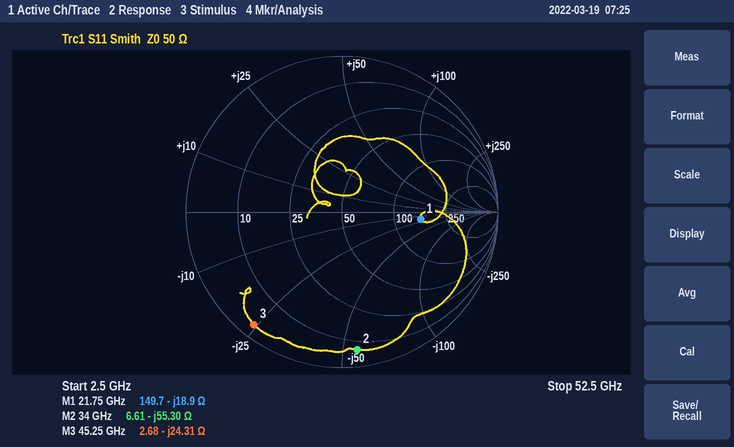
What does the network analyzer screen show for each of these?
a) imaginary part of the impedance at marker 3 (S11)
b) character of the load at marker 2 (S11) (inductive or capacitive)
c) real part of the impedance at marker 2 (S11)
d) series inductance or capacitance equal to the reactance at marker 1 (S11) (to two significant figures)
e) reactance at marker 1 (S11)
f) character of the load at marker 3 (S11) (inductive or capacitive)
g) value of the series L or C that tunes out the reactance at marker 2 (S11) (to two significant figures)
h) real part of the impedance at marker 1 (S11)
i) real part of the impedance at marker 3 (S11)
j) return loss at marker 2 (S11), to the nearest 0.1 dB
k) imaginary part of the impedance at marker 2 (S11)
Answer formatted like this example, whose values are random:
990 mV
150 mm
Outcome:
-24.31 Ω
capacitive
6.61 Ω
390 fF
-18.9 Ω
capacitive
260 pH
149.7 Ω
2.68 Ω
1.0 dB
-55.30 Ω
